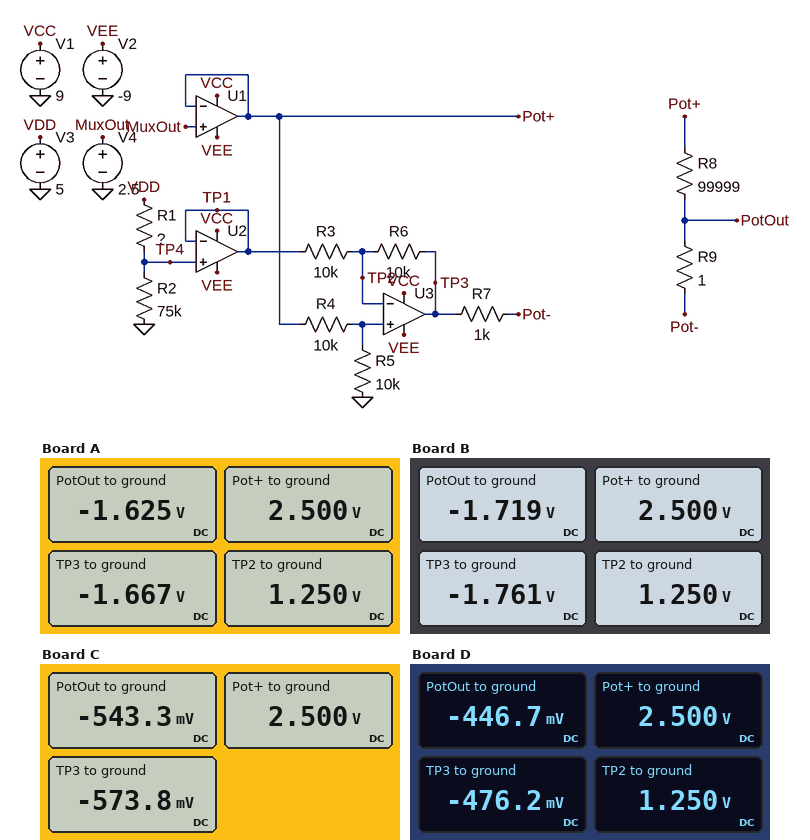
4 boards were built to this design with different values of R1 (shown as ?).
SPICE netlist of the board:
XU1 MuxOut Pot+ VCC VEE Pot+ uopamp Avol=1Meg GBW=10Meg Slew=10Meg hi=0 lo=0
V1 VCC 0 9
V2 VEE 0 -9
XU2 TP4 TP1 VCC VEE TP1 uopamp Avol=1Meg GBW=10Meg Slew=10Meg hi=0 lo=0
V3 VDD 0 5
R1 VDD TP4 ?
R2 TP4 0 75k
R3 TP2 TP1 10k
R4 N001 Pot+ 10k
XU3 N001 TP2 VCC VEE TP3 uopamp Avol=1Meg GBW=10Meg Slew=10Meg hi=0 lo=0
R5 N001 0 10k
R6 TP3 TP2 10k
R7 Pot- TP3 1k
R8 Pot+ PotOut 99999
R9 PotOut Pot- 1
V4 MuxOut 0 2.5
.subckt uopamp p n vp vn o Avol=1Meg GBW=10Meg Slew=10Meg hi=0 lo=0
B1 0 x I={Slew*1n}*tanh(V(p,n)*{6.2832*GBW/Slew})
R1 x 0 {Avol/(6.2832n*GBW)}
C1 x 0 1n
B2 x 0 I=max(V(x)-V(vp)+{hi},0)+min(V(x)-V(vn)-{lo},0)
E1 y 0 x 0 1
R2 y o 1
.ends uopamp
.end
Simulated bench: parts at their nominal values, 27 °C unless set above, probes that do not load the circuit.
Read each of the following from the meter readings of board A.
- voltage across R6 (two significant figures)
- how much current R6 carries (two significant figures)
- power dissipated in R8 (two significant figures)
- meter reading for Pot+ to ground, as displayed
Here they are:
2.9 V
290 µA
170 µW
2.500 V
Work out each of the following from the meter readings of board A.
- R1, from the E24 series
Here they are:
15 kΩ
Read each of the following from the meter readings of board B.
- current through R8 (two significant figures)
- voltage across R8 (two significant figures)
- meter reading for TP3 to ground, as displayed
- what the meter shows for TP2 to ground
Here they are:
42 µA
4.2 V
-1.761 V
1.250 V
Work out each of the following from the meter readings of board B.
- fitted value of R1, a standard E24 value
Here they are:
13 kΩ
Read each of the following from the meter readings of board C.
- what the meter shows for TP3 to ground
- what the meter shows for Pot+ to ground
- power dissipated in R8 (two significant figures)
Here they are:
-573.8 mV
2.500 V
93 µW
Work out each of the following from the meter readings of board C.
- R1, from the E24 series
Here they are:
47 kΩ
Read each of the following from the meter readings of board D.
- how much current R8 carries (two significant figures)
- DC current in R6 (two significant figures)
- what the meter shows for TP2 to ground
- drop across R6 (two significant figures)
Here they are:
29 µA
170 µA
1.250 V
1.7 V
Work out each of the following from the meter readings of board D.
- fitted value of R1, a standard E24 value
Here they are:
51 kΩ
